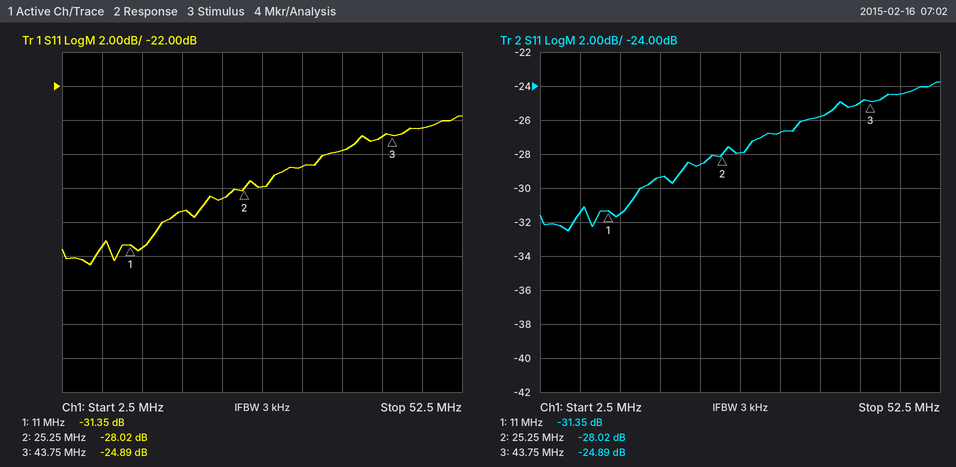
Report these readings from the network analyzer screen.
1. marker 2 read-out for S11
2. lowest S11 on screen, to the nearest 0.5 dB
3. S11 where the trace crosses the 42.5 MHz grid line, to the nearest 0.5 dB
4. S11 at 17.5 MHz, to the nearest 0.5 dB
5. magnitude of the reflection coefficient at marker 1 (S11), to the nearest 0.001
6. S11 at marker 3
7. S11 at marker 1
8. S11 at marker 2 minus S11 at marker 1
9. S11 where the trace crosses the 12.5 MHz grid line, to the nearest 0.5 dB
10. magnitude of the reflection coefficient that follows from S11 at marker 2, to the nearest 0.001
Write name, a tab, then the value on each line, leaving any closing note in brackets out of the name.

marker 2 read-out for S11	-28.02 dB
lowest S11 on screen, to the nearest 0.5 dB	-32.5 dB
S11 where the trace crosses the 42.5 MHz grid line, to the nearest 0.5 dB	-25.0 dB
S11 at 17.5 MHz, to the nearest 0.5 dB	-29.5 dB
magnitude of the reflection coefficient at marker 1 (S11), to the nearest 0.001	0.027
S11 at marker 3	-24.89 dB
S11 at marker 1	-31.35 dB
S11 at marker 2 minus S11 at marker 1	3.33 dB
S11 where the trace crosses the 12.5 MHz grid line, to the nearest 0.5 dB	-31.5 dB
magnitude of the reflection coefficient that follows from S11 at marker 2, to the nearest 0.001	0.040
